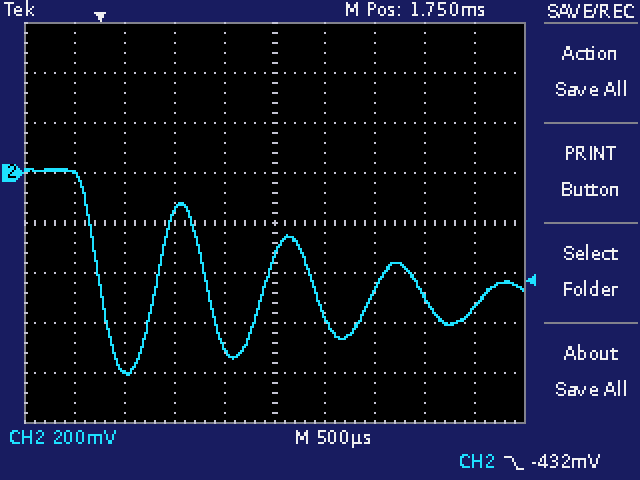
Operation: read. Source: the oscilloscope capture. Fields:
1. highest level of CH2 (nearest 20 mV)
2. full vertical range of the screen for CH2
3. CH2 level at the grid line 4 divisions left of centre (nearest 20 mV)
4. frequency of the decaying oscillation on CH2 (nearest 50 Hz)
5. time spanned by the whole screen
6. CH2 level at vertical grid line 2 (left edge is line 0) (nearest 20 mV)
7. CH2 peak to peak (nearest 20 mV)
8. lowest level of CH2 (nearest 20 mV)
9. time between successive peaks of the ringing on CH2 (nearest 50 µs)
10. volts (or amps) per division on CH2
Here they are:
20 mV
1.6 V
0 mV
950 Hz
5 ms
-800 mV
820 mV
-800 mV
1.05 ms
200 mV
